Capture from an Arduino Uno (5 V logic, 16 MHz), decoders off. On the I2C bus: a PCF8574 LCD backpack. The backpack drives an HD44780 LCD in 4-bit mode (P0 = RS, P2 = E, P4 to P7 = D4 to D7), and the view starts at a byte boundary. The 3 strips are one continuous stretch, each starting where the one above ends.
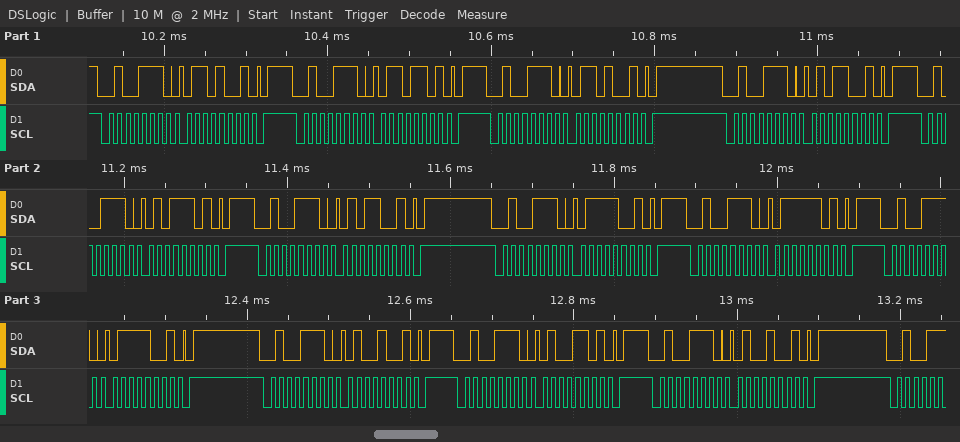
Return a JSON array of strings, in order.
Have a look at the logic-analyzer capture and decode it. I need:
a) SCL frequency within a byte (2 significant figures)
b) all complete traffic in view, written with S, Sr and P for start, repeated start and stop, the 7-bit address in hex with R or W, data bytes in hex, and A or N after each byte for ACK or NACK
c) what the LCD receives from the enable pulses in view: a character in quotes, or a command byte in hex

["100 kHz", "S 27W A 69 A P S 27W A 6D A P S 27W A 69 A P S 27W A 59 A P S 27W A 5D A P S 27W A 59 A P S 27W A 79 A P S 27W A 7D A P S 27W A 79 A P S 27W A 49 A P S 27W A 4D A P S 27W A 49 A P", "'e' 't'"]
